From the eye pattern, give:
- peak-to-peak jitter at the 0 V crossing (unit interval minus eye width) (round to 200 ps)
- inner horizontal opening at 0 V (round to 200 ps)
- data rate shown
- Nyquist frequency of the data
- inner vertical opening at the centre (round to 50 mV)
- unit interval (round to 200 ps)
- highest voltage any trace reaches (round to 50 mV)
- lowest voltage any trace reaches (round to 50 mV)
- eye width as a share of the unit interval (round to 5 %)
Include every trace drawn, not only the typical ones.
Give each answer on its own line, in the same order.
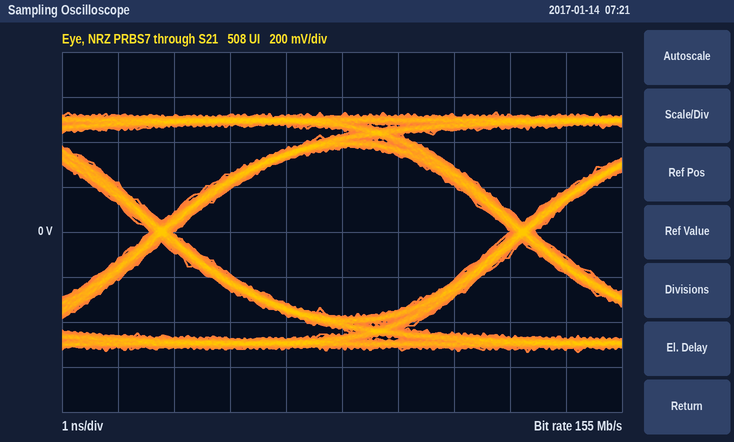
400 ps
6.0 ns
155 Mb/s
77.5 MHz
750 mV
6.4 ns
550 mV
-550 mV
95 %
